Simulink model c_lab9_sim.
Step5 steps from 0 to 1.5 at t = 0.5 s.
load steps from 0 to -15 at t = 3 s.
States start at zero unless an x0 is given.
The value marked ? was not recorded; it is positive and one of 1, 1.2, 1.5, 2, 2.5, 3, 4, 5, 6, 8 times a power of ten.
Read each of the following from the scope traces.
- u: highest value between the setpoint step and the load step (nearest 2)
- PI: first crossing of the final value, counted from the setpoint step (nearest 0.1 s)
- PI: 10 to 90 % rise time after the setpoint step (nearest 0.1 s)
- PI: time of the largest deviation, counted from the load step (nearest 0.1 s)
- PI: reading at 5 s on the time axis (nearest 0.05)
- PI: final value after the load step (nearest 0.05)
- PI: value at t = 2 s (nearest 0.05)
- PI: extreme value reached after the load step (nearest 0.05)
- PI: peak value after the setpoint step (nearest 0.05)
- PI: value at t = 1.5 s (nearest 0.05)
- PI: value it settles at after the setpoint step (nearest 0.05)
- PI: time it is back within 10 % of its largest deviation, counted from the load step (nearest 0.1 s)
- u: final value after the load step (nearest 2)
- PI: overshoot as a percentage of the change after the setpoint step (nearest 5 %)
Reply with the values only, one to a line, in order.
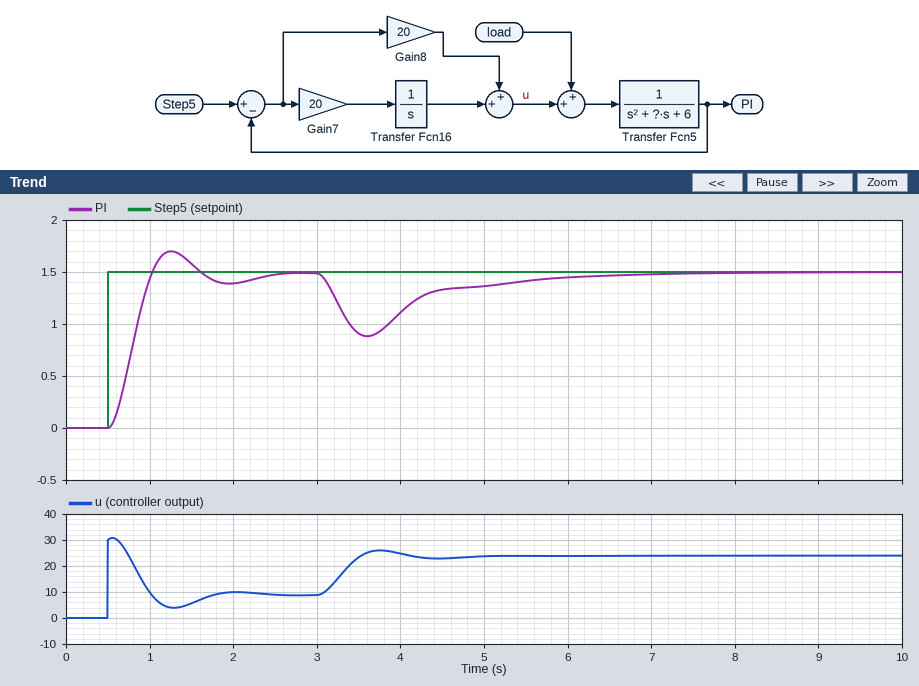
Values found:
30
0.5 s
0.4 s
0.6 s
1.35
1.50
1.40
0.90
1.70
1.60
1.50
2.8 s
24
15 %
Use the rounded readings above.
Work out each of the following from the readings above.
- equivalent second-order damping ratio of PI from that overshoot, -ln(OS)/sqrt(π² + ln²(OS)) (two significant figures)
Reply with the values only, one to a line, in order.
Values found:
0.52
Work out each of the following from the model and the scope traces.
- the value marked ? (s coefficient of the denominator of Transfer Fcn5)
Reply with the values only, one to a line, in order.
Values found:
5
